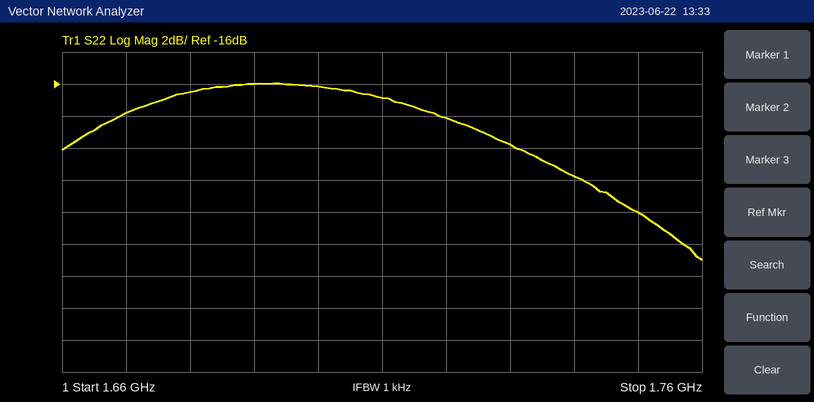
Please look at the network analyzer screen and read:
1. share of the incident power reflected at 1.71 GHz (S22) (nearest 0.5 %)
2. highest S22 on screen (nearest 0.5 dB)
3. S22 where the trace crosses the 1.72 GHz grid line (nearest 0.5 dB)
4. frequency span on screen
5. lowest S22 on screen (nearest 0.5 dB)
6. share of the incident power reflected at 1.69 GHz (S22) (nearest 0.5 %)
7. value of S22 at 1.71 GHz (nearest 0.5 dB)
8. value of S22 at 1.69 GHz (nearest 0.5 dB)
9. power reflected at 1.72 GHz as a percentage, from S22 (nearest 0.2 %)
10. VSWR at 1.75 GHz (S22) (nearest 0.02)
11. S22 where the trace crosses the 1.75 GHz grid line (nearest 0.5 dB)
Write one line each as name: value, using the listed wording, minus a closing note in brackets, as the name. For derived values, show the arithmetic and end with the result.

share of the incident power reflected at 1.71 GHz (S22): 10^(-17/10) ≈ 2.0 %
highest S22 on screen: -16.0 dB
S22 where the trace crosses the 1.72 GHz grid line: -18.0 dB
frequency span on screen: 100 MHz
lowest S22 on screen: -27.0 dB
share of the incident power reflected at 1.69 GHz (S22): 10^(-16/10) ≈ 2.5 %
value of S22 at 1.71 GHz: -17.0 dB
value of S22 at 1.69 GHz: -16.0 dB
power reflected at 1.72 GHz as a percentage, from S22: 10^(-18/10) ≈ 1.6 %
VSWR at 1.75 GHz (S22): |Γ| = 10^(-24/20) = 0.0631; VSWR = (1 + 0.0631)/(1 − 0.0631) ≈ 1.13, so 1.14 to the nearest 0.02
S22 where the trace crosses the 1.75 GHz grid line: -24.0 dB
